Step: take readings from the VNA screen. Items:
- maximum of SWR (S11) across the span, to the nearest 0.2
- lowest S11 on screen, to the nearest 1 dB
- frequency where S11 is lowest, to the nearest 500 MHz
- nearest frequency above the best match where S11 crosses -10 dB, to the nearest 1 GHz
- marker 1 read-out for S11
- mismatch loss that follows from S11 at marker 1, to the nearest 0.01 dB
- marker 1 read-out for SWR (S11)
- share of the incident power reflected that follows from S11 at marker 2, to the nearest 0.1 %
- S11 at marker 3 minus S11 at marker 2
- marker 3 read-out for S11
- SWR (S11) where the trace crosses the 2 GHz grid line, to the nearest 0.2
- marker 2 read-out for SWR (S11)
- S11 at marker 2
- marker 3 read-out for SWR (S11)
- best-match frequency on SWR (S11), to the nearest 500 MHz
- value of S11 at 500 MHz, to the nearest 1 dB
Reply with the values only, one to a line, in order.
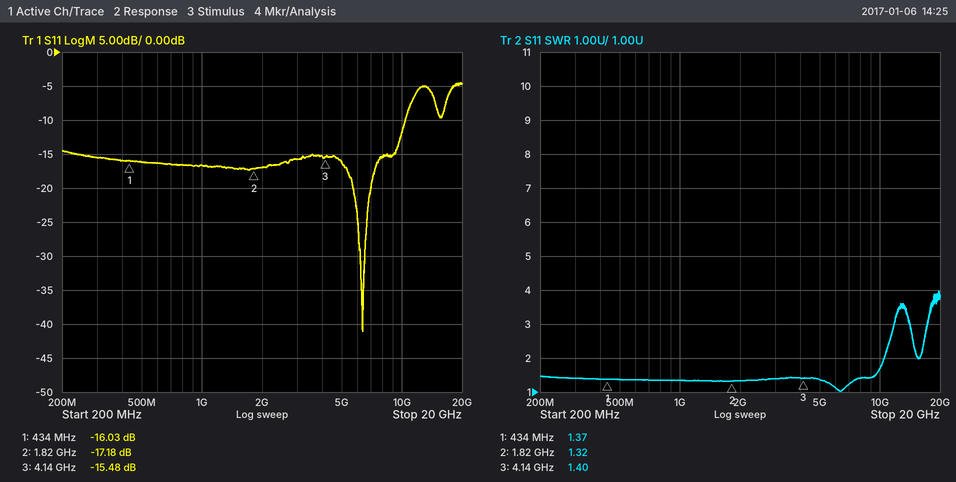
4.0
-41 dB
6.5 GHz
10 GHz
-16.03 dB
0.11 dB
1.37
1.9 %
1.70 dB
-15.48 dB
1.4
1.32
-17.18 dB
1.40
6.5 GHz
-16 dB
